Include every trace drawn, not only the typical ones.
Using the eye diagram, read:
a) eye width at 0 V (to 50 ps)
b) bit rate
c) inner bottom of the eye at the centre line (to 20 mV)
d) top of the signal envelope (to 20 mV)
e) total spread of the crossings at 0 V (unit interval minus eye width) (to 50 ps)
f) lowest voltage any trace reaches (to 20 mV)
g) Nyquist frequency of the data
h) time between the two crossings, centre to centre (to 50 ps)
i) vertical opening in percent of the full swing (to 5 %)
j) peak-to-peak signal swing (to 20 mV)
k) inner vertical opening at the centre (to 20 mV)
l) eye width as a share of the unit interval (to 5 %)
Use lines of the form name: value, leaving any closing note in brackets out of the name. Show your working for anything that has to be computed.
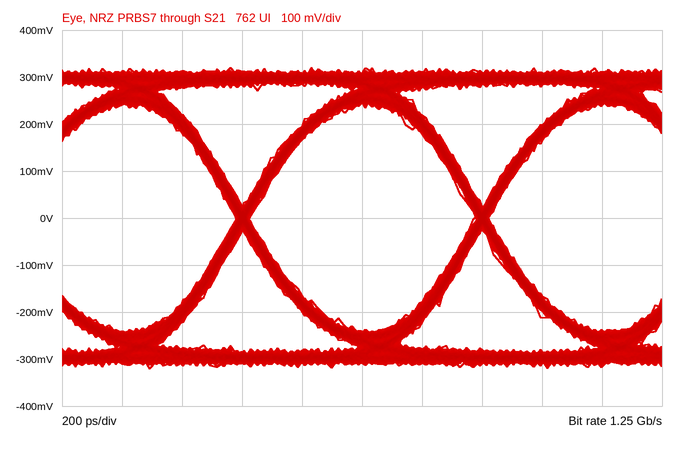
eye width at 0 V: 750 ps
bit rate: 1.25 Gb/s
inner bottom of the eye at the centre line: -240 mV
top of the signal envelope: 320 mV
total spread of the crossings at 0 V (unit interval minus eye width): 50 ps
lowest voltage any trace reaches: -320 mV
Nyquist frequency of the data: 625 MHz
time between the two crossings, centre to centre: 800 ps
vertical opening in percent of the full swing: 480 mV / 640 mV ≈ 75 %
peak-to-peak signal swing: 640 mV
inner vertical opening at the centre: 480 mV
eye width as a share of the unit interval: 750 ps / 800 ps ≈ 93.7 %, so 95 % to the nearest 5 %
